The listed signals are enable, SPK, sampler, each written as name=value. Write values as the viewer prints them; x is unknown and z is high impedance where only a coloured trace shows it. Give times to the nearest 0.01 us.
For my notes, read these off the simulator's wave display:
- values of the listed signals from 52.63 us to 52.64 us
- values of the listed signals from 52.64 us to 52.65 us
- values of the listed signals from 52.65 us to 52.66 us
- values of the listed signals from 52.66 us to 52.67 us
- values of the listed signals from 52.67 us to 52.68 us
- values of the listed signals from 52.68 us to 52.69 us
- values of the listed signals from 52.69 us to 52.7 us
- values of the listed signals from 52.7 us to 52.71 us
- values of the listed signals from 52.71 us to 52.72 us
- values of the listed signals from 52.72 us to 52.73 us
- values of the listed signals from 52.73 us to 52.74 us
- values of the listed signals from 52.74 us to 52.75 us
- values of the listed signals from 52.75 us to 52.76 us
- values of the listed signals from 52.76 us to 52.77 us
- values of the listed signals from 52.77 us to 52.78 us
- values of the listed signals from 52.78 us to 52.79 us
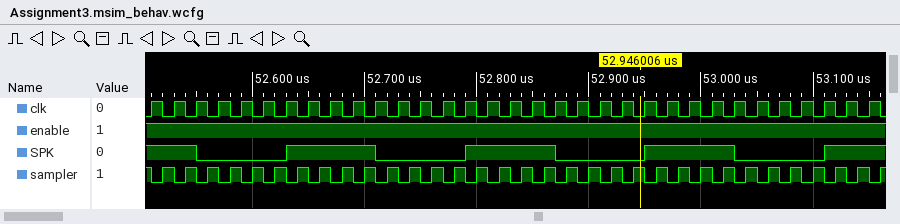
enable=1, SPK=1, sampler=0
enable=1, SPK=1, sampler=1
enable=1, SPK=1, sampler=0
enable=1, SPK=1, sampler=1
enable=1, SPK=1, sampler=0
enable=1, SPK=1, sampler=1
enable=1, SPK=1, sampler=0
enable=1, SPK=1, sampler=1
enable=1, SPK=0, sampler=0
enable=1, SPK=0, sampler=1
enable=1, SPK=0, sampler=0
enable=1, SPK=0, sampler=1
enable=1, SPK=0, sampler=0
enable=1, SPK=0, sampler=1
enable=1, SPK=0, sampler=0
enable=1, SPK=0, sampler=1
